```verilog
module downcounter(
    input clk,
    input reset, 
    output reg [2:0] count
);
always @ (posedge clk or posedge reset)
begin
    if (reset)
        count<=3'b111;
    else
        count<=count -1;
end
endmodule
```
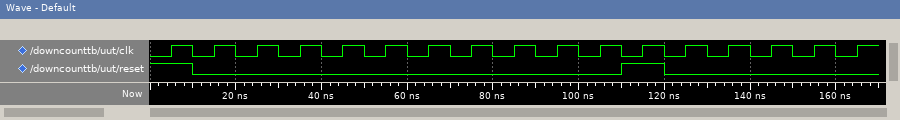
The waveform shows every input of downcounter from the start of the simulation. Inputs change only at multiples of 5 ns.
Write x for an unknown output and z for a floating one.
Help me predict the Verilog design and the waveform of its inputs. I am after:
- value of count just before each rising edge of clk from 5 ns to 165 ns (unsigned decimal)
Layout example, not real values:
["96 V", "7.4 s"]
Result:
["7, 7, 6, 5, 4, 3, 2, 1, 0, 7, 6, 7, 7, 6, 5, 4, 3"]
